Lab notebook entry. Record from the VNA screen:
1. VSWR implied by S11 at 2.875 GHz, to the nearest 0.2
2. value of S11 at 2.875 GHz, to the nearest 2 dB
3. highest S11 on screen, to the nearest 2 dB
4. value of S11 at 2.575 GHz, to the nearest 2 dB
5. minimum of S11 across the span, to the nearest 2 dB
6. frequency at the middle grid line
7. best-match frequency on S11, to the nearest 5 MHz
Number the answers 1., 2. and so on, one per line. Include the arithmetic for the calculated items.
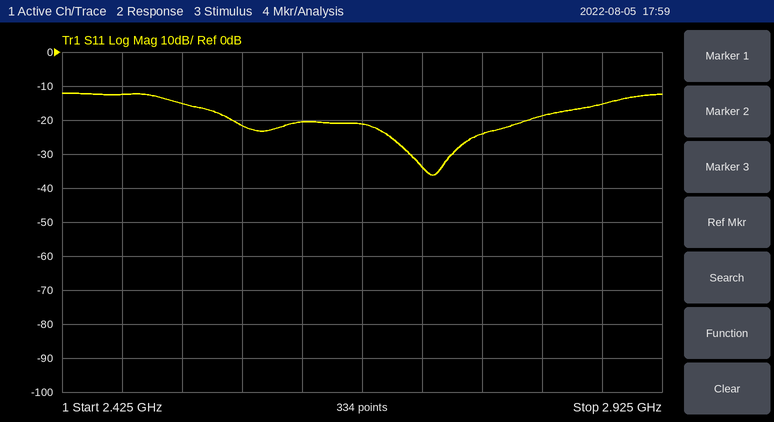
1. |Γ| = 10^(-16/20) = 0.1585; VSWR = (1 + 0.1585)/(1 − 0.1585) ≈ 1.4
2. -16 dB
3. -12 dB
4. -22 dB
5. -36 dB
6. 2.675 GHz
7. 2.735 GHz
